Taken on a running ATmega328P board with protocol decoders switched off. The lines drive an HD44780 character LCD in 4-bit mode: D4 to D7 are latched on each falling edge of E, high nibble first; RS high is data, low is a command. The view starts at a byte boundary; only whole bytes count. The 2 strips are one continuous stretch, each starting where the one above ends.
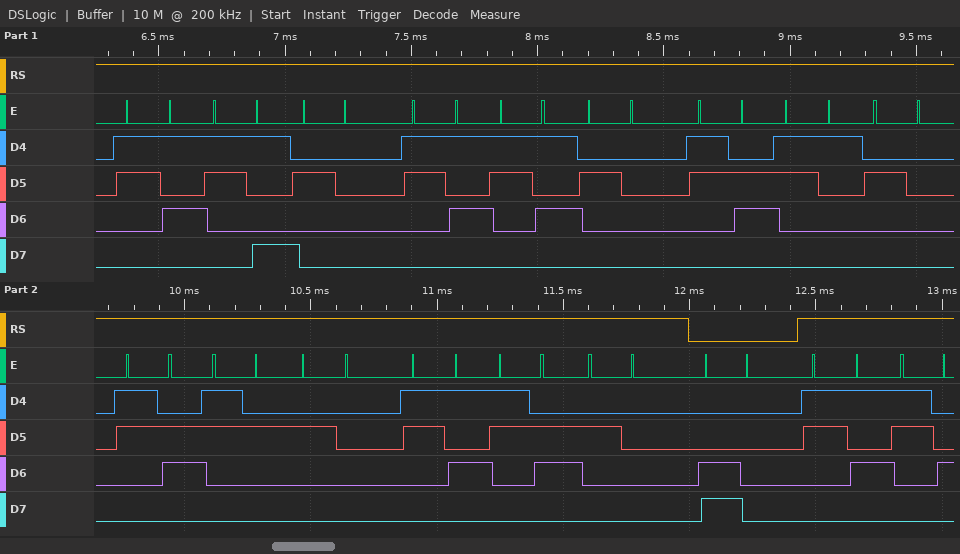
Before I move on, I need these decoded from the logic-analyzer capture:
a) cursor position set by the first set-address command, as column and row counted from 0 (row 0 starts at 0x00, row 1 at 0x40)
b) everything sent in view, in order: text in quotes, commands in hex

column 0, row 1
"59 55 61 62 56 " 0xC0 "54"
